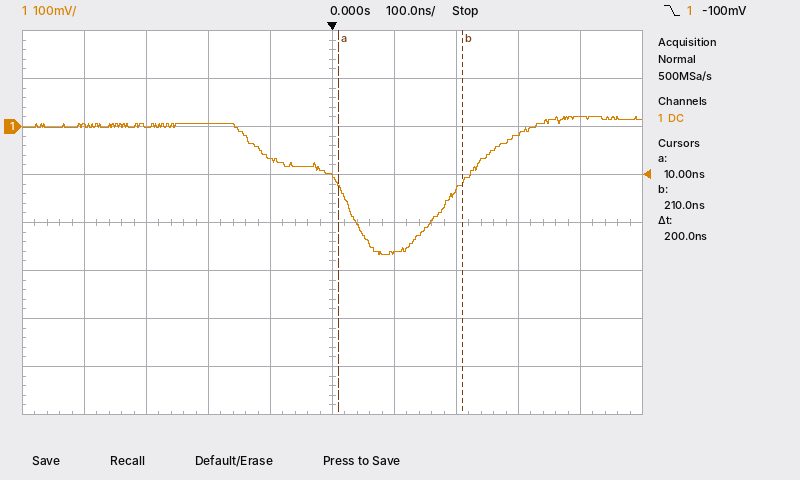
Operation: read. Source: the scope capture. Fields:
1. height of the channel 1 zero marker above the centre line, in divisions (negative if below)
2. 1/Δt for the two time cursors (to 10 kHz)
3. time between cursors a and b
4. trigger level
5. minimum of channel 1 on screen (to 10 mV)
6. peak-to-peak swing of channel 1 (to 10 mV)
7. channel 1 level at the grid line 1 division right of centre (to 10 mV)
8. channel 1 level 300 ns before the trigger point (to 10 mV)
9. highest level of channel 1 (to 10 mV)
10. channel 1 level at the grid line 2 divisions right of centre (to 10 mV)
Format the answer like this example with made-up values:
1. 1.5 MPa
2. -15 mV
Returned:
1. +2.0 div
2. 5.00 MHz
3. 200 ns
4. -100 mV
5. -270 mV
6. 290 mV
7. -260 mV
8. 0 mV
9. 20 mV
10. -130 mV
